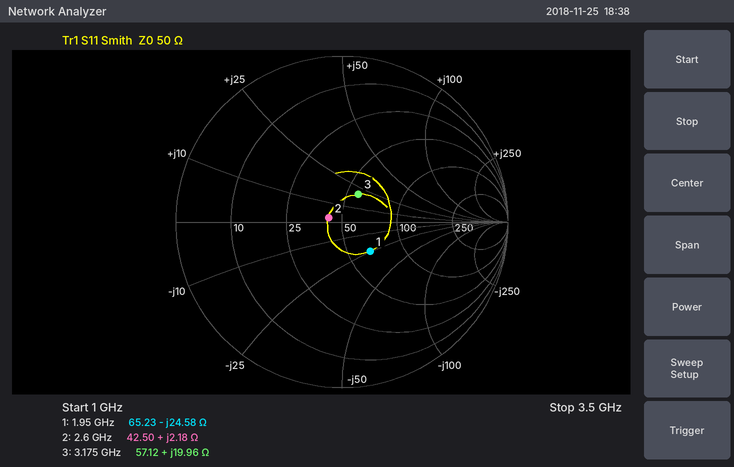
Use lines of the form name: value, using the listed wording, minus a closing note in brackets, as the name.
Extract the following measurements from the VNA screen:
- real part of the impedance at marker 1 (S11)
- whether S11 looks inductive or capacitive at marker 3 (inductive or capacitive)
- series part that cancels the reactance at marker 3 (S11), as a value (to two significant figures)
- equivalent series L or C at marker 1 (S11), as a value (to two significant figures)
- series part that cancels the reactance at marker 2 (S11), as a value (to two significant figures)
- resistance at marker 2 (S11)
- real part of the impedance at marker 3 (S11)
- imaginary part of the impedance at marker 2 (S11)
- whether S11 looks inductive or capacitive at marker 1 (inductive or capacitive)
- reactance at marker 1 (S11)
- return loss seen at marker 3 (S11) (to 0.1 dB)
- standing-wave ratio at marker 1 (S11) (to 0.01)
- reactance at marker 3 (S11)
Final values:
real part of the impedance at marker 1: 65.23 Ω
whether S11 looks inductive or capacitive at marker 3: inductive
series part that cancels the reactance at marker 3 (S11), as a value: 2.5 pF
equivalent series L or C at marker 1 (S11), as a value: 3.3 pF
series part that cancels the reactance at marker 2 (S11), as a value: 28 pF
resistance at marker 2: 42.50 Ω
real part of the impedance at marker 3: 57.12 Ω
imaginary part of the impedance at marker 2: +2.18 Ω
whether S11 looks inductive or capacitive at marker 1: capacitive
reactance at marker 1: -24.58 Ω
return loss seen at marker 3 (S11): 14.2 dB
standing-wave ratio at marker 1 (S11): 1.65
reactance at marker 3: +19.96 Ω
